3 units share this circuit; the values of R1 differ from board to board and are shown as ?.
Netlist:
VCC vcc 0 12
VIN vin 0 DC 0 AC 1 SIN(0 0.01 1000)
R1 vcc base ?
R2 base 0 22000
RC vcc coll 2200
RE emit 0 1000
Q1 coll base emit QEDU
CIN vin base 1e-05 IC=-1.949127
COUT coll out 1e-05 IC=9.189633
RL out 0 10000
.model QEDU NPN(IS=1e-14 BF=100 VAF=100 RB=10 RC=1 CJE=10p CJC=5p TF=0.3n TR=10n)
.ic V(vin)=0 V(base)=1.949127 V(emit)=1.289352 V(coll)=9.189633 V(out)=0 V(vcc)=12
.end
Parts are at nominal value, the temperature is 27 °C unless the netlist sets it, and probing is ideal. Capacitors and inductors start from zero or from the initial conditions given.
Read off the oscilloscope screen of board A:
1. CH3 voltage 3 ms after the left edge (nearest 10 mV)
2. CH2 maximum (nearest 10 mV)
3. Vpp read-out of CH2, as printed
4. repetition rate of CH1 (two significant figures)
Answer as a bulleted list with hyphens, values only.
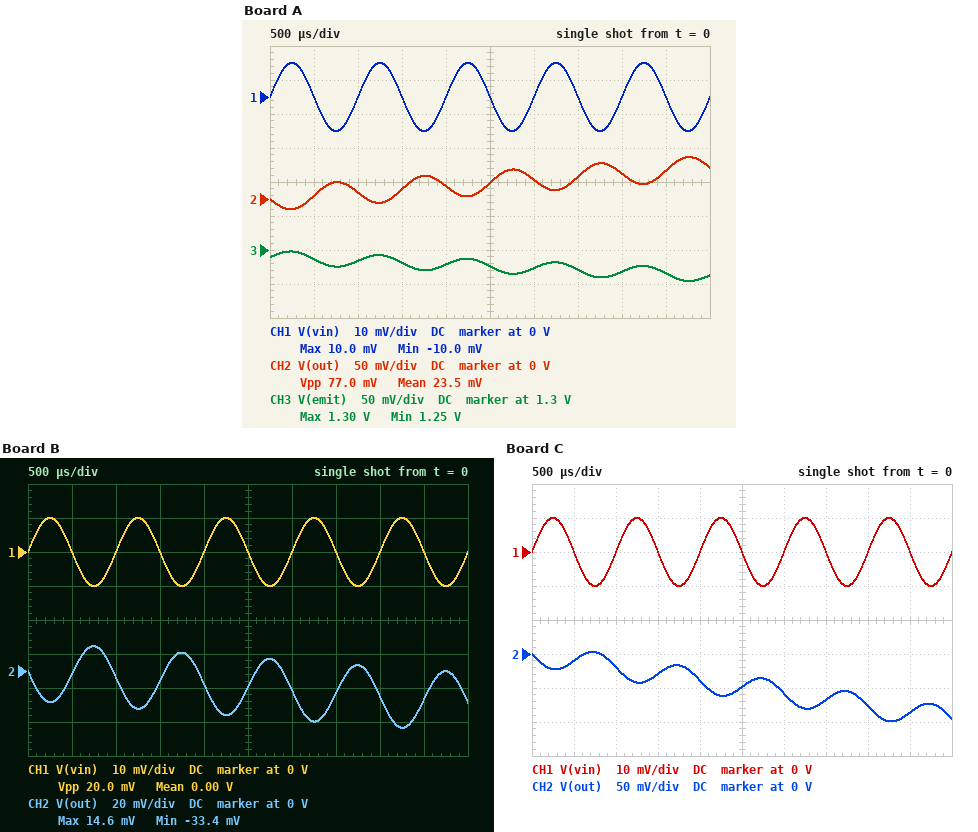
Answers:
- 1.27 V
- 60 mV
- 77.0 mV
- 1.0 kHz
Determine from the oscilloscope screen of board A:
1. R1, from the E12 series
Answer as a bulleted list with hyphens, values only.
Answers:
- 220 kΩ
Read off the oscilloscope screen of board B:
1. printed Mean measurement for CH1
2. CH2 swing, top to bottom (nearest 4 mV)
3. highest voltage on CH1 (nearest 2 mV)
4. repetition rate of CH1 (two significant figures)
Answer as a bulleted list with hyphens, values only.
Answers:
- 0.00 V
- 48 mV
- 10 mV
- 1.0 kHz
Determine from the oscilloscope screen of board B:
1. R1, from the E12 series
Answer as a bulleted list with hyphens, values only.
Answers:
- 82 kΩ
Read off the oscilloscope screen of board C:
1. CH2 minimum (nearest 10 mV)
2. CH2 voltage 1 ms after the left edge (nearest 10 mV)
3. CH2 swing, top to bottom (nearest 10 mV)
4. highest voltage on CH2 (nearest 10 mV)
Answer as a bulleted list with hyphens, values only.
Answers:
- -100 mV
- -20 mV
- 100 mV
- 0 V
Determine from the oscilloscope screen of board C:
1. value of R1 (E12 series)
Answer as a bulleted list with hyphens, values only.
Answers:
- 47 kΩ
